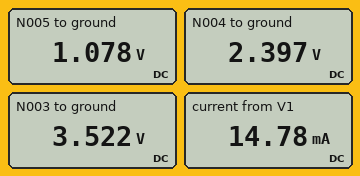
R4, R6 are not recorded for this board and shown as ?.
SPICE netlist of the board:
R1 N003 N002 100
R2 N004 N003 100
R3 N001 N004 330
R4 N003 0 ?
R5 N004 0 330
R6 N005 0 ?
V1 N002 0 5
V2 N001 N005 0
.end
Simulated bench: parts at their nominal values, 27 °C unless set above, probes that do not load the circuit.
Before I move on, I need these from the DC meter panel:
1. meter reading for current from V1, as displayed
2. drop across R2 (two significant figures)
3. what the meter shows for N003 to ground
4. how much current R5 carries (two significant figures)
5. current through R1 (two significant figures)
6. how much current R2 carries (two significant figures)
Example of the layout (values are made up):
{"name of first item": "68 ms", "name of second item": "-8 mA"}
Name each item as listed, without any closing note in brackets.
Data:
{"meter reading for current from V1, as displayed": "14.78 mA", "drop across R2": "1.1 V", "what the meter shows for N003 to ground": "3.522 V", "how much current R5 carries": "7.3 mA", "current through R1": "15 mA", "how much current R2 carries": "11 mA"}
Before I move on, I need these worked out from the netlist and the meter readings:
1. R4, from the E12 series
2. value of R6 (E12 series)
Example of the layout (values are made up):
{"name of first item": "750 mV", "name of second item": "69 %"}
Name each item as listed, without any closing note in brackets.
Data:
{"R4, from the E12 series": "1 kΩ", "value of R6": "270 Ω"}
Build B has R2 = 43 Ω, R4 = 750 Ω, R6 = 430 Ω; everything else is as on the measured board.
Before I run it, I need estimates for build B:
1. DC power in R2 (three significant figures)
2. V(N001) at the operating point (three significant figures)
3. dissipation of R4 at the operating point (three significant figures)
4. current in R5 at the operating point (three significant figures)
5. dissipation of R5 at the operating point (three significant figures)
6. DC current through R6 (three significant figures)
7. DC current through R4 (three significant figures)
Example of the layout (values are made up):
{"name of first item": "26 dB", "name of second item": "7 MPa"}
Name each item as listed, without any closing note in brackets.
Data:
{"DC power in R2": "6.41 mW", "V(N001) at the operating point": "1.59 V", "dissipation of R4 at the operating point": "14.8 mW", "current in R5 at the operating point": "8.51 mA", "dissipation of R5 at the operating point": "23.9 mW", "DC current through R6": "3.70 mA", "DC current through R4": "4.45 mA"}
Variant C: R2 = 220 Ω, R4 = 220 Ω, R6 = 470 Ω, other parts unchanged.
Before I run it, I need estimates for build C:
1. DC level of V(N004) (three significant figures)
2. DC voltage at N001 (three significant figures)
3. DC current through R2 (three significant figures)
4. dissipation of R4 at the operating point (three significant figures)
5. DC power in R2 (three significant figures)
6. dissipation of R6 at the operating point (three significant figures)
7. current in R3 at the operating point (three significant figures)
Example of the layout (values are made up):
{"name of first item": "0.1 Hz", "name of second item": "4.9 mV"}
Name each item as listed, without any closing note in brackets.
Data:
{"DC level of V(N004)": "1.54 V", "DC voltage at N001": "903 mV", "DC current through R2": "6.58 mA", "dissipation of R4 at the operating point": "40.5 mW", "DC power in R2": "9.53 mW", "dissipation of R6 at the operating point": "1.74 mW", "current in R3 at the operating point": "1.92 mA"}
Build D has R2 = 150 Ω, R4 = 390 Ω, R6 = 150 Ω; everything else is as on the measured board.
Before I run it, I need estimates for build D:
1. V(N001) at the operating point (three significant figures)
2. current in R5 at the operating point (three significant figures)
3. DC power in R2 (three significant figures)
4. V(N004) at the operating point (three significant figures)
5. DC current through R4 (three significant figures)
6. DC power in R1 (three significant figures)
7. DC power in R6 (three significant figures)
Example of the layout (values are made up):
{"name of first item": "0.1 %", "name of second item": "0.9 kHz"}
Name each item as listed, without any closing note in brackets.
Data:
{"V(N001) at the operating point": "572 mV", "current in R5 at the operating point": "5.55 mA", "DC power in R2": "13.1 mW", "V(N004) at the operating point": "1.83 V", "DC current through R4": "8.29 mA", "DC power in R1": "31.2 mW", "DC power in R6": "2.18 mW"}
